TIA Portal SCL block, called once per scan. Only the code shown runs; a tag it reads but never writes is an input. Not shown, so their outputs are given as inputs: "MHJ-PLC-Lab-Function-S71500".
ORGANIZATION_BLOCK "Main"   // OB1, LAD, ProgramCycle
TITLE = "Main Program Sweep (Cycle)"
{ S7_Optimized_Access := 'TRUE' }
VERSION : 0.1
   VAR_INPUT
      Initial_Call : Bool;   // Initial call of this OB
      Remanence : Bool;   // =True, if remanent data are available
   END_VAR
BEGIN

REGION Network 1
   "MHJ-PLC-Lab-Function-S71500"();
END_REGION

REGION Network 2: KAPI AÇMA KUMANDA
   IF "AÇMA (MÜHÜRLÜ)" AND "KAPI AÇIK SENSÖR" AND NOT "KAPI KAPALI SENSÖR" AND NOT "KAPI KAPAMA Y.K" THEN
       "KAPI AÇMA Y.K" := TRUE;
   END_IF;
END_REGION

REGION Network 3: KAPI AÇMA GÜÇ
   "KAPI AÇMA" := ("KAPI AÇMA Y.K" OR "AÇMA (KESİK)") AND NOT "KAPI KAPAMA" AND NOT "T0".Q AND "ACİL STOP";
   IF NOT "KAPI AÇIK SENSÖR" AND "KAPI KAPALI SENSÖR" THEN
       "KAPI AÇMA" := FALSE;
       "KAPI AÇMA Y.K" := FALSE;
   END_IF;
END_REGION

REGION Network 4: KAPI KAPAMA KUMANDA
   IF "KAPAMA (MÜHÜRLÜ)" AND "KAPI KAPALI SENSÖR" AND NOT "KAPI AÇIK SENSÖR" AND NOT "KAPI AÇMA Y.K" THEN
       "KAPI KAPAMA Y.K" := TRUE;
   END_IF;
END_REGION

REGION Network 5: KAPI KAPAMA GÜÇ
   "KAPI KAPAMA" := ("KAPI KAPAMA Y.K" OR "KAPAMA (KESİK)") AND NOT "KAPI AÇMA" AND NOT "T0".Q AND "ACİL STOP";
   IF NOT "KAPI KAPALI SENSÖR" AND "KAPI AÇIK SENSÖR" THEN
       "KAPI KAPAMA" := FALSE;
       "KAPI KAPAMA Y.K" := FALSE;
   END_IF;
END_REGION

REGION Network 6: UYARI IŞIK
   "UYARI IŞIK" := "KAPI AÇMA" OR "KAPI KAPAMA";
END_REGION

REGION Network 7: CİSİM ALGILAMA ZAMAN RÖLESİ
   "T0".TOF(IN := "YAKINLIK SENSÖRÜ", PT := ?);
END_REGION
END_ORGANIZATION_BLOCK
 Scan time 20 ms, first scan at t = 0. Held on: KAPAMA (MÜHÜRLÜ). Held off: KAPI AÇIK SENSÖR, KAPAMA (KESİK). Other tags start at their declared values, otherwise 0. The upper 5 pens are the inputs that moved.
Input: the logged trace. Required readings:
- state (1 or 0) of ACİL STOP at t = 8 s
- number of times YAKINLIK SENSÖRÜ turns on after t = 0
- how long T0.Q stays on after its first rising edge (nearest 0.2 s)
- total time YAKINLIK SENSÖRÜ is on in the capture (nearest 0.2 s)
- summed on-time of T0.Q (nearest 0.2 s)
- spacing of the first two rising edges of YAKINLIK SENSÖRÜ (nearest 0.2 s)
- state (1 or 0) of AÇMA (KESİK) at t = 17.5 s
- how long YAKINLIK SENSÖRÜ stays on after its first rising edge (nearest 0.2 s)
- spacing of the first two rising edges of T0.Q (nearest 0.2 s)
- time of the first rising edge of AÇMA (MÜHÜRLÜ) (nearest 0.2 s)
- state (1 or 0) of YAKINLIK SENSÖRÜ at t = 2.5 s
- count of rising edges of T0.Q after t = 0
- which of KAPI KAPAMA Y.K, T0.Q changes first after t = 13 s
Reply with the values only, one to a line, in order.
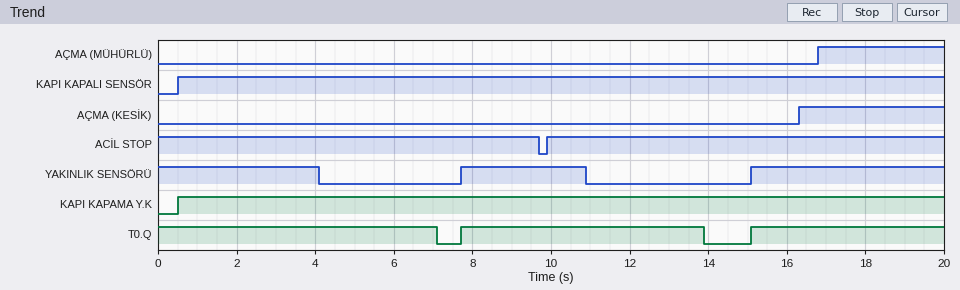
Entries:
1
2
6.2 s
12.2 s
18.2 s
7.4 s
1
3.2 s
7.4 s
16.8 s
1
2
T0.Q
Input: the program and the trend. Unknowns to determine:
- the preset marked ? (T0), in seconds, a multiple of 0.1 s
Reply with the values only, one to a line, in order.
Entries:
3.0 s
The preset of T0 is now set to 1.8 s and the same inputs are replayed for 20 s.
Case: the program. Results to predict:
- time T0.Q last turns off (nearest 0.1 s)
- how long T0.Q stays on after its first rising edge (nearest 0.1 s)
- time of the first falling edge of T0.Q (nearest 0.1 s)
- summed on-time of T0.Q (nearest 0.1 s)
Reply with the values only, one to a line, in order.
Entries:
12.7 s
5.0 s
5.9 s
15.8 s
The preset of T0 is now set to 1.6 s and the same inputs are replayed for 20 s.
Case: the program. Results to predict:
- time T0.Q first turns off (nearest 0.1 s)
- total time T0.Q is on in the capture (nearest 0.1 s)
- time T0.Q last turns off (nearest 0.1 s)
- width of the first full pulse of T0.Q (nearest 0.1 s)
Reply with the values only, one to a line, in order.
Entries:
5.7 s
15.4 s
12.5 s
4.8 s
